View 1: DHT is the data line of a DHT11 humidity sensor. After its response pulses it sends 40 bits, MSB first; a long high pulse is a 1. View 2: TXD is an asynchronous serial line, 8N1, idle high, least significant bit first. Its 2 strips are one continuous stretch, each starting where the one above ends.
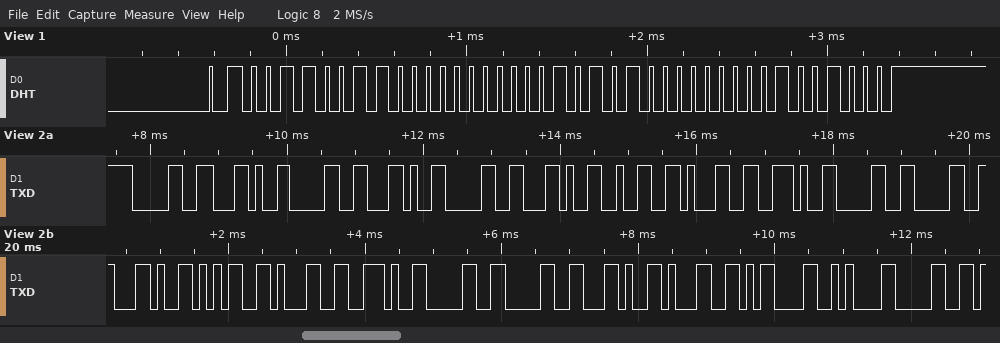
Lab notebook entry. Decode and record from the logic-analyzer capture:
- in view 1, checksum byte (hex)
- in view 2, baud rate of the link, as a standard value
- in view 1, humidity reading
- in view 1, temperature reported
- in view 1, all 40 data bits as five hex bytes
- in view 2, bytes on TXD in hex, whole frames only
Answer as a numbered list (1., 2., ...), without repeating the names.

1. 0x48
2. 9600 baud
3. 51 %
4. 21.0 °C
5. 33 00 15 00 48
6. 0x30 0x2C 0x30 0x2C 0x30 0x2C 0x32 0x31 0x2E 0x30 0x30 0x2C 0x35 0x31 0x2E 0x30 0x30 0x2C 0x31 0x0D 0x0A 0x30
